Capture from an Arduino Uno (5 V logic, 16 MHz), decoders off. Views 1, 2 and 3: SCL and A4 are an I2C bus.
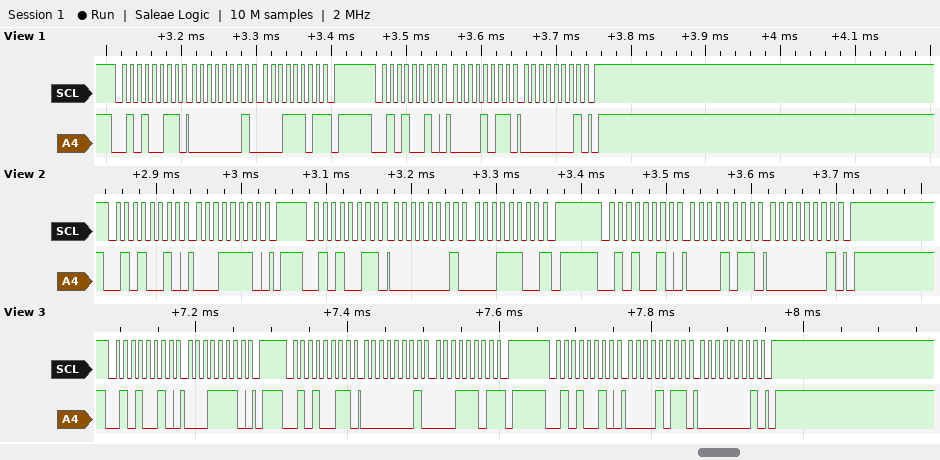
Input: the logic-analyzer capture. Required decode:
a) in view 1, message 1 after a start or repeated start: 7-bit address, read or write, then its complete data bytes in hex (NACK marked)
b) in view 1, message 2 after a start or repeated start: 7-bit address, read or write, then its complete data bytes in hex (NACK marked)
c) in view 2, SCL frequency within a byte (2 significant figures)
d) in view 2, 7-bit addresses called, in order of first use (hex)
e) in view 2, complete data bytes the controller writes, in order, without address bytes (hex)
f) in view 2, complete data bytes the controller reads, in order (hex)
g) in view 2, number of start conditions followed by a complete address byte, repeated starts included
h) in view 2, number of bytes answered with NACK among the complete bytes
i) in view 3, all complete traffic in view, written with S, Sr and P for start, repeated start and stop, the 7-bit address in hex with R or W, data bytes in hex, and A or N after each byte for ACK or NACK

0x29 read: 01 1D NACK
0x29 write: 0B 01
100 kHz
0x29
1E 0B 01
01 1C
3
1
S 29W A 1E A P S 29R A 01 A 1D N P S 29W A 0B A 01 A P
